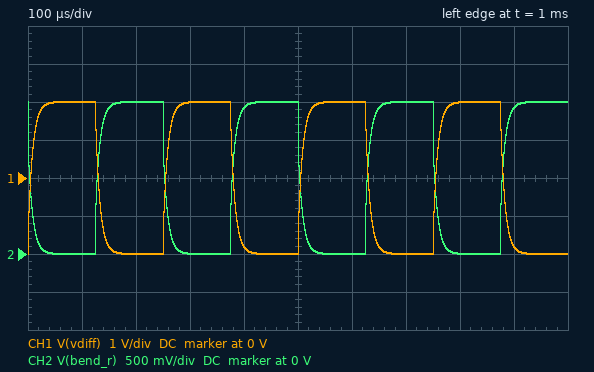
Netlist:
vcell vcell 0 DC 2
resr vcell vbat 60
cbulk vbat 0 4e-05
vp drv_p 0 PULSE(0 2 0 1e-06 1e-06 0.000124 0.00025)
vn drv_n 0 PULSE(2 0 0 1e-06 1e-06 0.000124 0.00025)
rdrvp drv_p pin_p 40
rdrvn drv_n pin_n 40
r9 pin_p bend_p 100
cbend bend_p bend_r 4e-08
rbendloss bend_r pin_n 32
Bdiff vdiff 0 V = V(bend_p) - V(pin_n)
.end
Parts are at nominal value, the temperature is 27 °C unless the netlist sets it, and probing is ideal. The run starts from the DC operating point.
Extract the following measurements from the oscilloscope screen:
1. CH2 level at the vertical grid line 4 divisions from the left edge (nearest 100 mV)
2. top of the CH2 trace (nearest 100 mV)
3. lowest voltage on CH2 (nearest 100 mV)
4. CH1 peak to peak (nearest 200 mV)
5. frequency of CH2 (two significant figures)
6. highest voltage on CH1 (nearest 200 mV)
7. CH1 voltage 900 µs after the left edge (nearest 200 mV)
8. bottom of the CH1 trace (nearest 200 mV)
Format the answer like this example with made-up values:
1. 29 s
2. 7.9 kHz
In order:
1. 1.9 V
2. 2.0 V
3. 0 V
4. 4.0 V
5. 4.0 kHz
6. 2.0 V
7. -1.8 V
8. -2.0 V
